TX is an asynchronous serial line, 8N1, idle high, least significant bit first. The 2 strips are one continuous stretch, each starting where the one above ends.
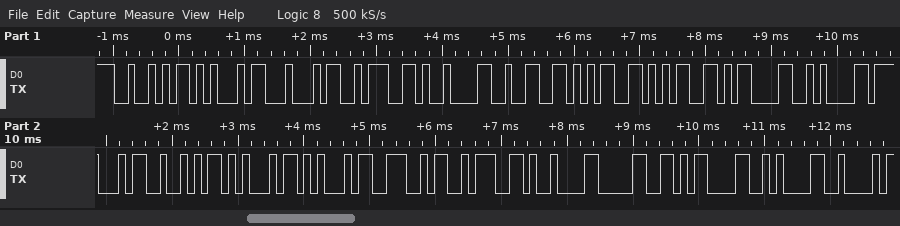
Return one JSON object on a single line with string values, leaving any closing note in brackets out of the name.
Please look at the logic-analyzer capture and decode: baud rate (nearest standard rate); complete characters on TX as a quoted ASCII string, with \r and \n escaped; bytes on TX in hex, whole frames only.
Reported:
{"baud rate": "9600 baud", "complete characters on TX as a quoted ASCII string, with \\r and \\n escaped": "\"RED:\\t255\\r\\nGREEN:\\t0\\r\\nB\"", "bytes on TX in hex, whole frames only": "0x52 0x45 0x44 0x3A 0x09 0x32 0x35 0x35 0x0D 0x0A 0x47 0x52 0x45 0x45 0x4E 0x3A 0x09 0x30 0x0D 0x0A 0x42"}
